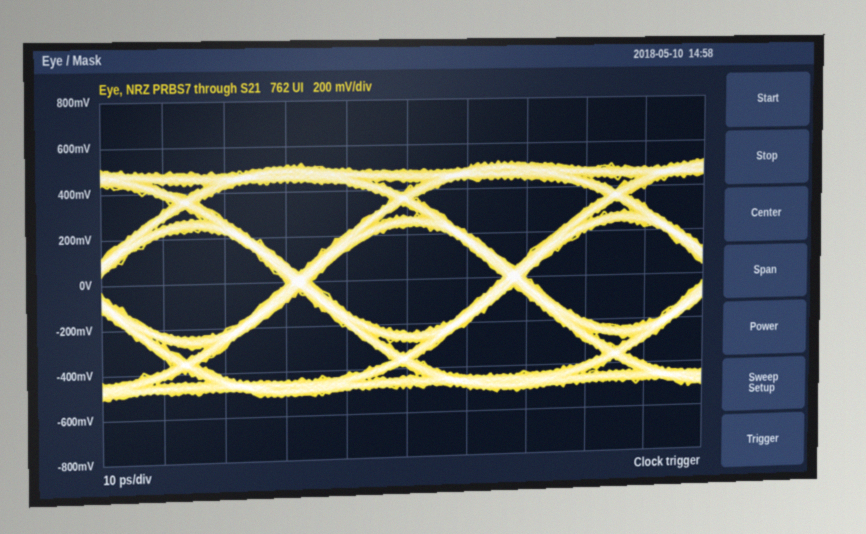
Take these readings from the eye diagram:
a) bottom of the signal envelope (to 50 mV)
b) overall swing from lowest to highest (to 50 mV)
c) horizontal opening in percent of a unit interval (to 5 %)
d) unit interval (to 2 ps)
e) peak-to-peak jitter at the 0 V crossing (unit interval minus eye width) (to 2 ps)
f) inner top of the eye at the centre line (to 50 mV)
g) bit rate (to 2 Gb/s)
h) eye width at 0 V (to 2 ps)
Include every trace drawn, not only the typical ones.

-500 mV
1.05 V
90 %
36 ps
4 ps
250 mV
28 Gb/s
32 ps
